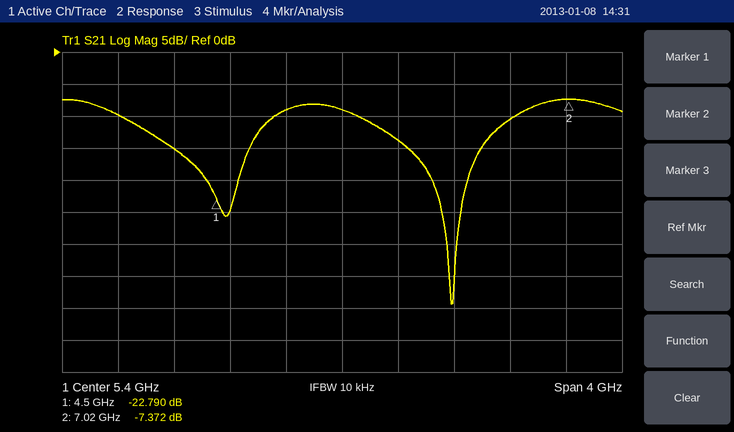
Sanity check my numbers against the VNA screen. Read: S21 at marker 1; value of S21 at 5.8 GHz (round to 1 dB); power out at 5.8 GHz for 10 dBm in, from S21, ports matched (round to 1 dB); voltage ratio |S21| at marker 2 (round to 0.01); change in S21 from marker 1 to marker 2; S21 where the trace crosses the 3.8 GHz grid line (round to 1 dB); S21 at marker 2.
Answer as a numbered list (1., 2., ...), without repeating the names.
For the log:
1. -22.790 dB
2. -14 dB
3. -4 dBm
4. 0.43
5. 15.418 dB
6. -10 dB
7. -7.372 dB
